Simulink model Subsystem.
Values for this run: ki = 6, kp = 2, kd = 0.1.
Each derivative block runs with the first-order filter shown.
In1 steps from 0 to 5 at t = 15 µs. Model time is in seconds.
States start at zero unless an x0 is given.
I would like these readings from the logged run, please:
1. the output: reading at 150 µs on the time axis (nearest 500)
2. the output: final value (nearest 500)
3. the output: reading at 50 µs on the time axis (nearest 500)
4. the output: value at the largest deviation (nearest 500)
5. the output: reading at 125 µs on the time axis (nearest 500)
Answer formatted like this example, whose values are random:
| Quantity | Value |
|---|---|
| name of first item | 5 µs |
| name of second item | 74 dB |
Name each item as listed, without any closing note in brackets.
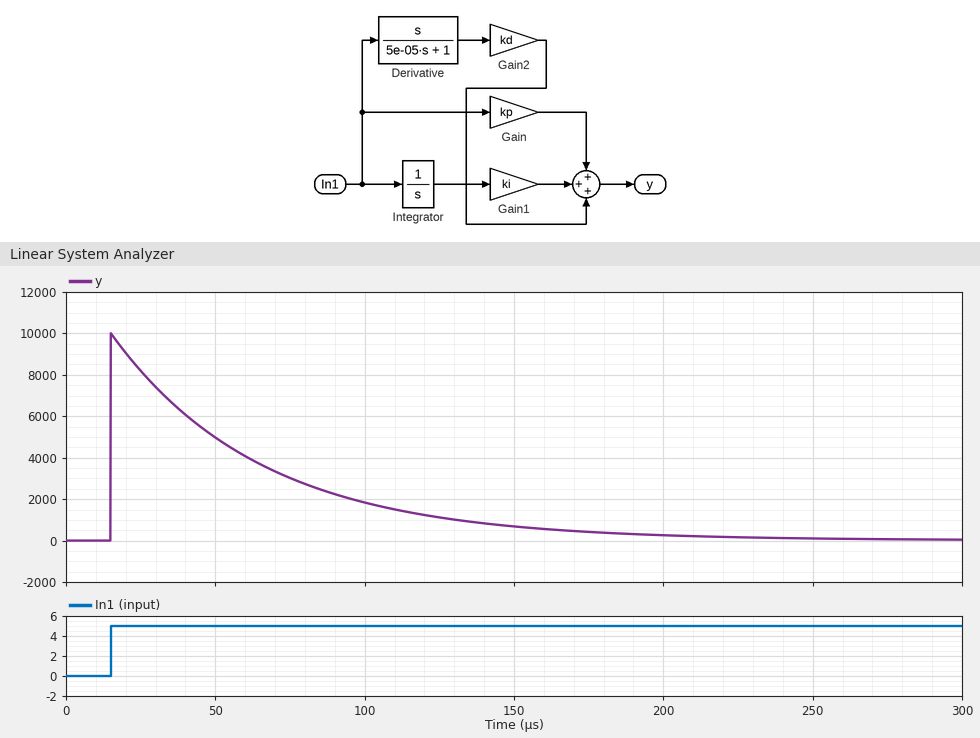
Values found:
| Quantity | Value |
|---|---|
| the output: reading at 150 µs on the time axis | 500 |
| the output: final value | 0 |
| the output: reading at 50 µs on the time axis | 5000 |
| the output: value at the largest deviation | 10000 |
| the output: reading at 125 µs on the time axis | 1000 |
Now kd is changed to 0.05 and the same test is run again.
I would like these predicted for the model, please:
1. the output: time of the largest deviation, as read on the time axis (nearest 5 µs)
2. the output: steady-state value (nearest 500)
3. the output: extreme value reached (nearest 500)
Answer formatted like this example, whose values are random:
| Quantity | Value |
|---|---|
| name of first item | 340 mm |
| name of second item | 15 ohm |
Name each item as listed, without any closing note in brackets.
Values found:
| Quantity | Value |
|---|---|
| the output: time of the largest deviation, as read on the time axis | 15 µs |
| the output: steady-state value | 0 |
| the output: extreme value reached | 5000 |
